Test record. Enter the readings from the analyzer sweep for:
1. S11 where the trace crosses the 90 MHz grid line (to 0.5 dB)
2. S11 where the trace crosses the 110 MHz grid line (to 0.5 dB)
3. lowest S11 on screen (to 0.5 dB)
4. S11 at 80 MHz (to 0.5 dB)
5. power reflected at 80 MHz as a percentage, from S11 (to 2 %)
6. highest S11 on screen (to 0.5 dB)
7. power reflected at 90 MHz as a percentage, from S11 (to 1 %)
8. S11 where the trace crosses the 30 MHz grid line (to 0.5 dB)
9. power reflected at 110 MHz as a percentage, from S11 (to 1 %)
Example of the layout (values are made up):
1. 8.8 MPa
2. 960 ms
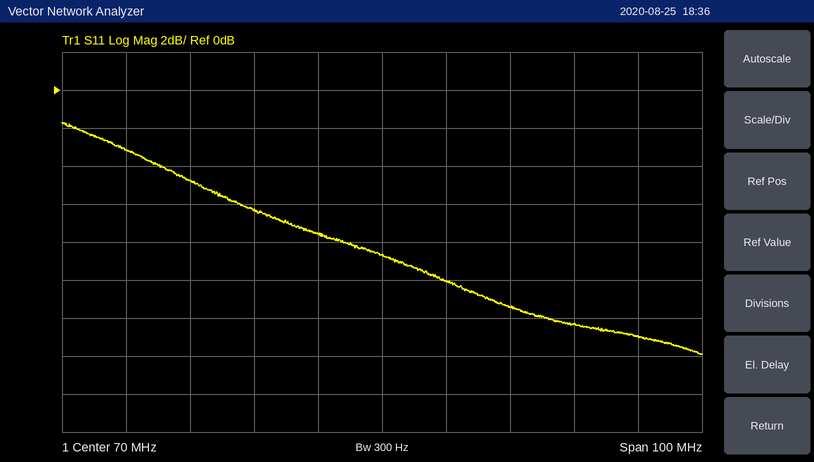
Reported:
1. -11.5 dB
2. -13.0 dB
3. -14.0 dB
4. -10.0 dB
5. 10 %
6. -1.5 dB
7. 7 %
8. -3.0 dB
9. 5 %
